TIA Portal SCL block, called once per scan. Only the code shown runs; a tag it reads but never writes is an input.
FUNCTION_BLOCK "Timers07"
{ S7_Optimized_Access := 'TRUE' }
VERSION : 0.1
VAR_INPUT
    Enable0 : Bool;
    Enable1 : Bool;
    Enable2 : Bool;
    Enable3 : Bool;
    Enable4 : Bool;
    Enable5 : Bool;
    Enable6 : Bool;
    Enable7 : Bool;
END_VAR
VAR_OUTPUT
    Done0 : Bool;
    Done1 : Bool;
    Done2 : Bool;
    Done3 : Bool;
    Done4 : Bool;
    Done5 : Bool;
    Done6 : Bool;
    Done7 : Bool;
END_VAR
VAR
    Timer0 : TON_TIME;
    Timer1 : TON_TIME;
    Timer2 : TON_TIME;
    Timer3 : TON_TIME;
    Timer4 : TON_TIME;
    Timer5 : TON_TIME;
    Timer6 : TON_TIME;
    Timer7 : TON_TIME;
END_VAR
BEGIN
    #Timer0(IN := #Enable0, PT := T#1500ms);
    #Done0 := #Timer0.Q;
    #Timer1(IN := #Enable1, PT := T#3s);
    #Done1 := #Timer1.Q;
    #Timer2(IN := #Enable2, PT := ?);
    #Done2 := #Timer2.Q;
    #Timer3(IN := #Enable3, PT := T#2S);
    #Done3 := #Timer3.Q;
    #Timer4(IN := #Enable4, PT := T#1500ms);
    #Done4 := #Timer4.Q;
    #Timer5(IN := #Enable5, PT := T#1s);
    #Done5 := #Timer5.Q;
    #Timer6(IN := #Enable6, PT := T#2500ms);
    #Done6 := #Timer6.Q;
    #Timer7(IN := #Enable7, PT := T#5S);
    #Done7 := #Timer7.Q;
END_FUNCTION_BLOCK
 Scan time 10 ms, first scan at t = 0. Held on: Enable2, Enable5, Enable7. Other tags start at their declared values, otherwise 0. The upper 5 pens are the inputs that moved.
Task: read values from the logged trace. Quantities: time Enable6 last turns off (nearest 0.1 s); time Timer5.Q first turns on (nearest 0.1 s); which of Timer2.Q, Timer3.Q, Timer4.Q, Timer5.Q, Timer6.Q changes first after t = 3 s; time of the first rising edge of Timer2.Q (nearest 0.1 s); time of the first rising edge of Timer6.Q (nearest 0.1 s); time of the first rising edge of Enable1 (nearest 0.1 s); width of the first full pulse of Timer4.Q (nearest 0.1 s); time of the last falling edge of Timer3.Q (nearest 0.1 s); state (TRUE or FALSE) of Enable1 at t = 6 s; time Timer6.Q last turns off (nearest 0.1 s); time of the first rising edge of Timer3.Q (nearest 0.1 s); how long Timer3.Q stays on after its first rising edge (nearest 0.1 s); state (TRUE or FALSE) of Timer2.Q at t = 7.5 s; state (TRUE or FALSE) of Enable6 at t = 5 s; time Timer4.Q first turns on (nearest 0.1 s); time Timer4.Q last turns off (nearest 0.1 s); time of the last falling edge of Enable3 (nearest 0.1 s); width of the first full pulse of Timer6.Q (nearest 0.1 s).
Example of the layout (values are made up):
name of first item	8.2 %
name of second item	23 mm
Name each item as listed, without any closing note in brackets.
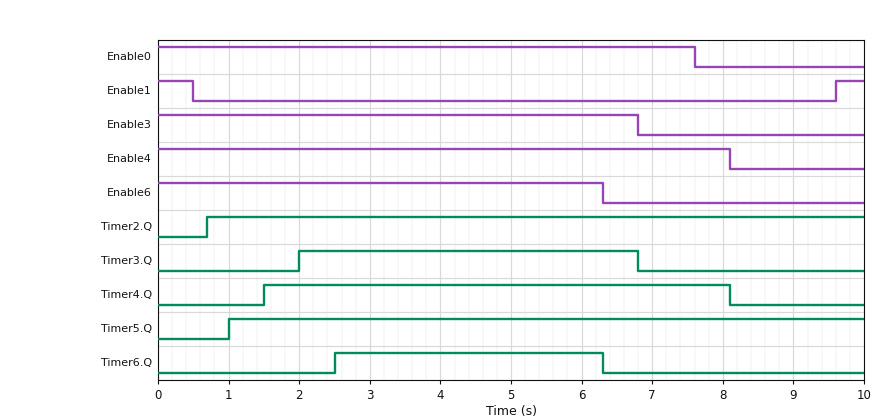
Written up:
time Enable6 last turns off	6.3 s
time Timer5.Q first turns on	1.0 s
which of Timer2.Q, Timer3.Q, Timer4.Q, Timer5.Q, Timer6.Q changes first after t = 3 s	Timer6.Q
time of the first rising edge of Timer2.Q	0.7 s
time of the first rising edge of Timer6.Q	2.5 s
time of the first rising edge of Enable1	9.6 s
width of the first full pulse of Timer4.Q	6.6 s
time of the last falling edge of Timer3.Q	6.8 s
state (TRUE or FALSE) of Enable1 at t = 6 s	FALSE
time Timer6.Q last turns off	6.3 s
time of the first rising edge of Timer3.Q	2.0 s
how long Timer3.Q stays on after its first rising edge	4.8 s
state (TRUE or FALSE) of Timer2.Q at t = 7.5 s	TRUE
state (TRUE or FALSE) of Enable6 at t = 5 s	TRUE
time Timer4.Q first turns on	1.5 s
time Timer4.Q last turns off	8.1 s
time of the last falling edge of Enable3	6.8 s
width of the first full pulse of Timer6.Q	3.8 s
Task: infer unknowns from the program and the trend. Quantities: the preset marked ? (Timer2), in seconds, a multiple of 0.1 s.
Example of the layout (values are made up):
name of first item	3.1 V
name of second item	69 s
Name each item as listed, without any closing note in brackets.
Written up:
the preset marked ? (Timer2), in seconds, a multiple of 0.1 s	0.7 s
